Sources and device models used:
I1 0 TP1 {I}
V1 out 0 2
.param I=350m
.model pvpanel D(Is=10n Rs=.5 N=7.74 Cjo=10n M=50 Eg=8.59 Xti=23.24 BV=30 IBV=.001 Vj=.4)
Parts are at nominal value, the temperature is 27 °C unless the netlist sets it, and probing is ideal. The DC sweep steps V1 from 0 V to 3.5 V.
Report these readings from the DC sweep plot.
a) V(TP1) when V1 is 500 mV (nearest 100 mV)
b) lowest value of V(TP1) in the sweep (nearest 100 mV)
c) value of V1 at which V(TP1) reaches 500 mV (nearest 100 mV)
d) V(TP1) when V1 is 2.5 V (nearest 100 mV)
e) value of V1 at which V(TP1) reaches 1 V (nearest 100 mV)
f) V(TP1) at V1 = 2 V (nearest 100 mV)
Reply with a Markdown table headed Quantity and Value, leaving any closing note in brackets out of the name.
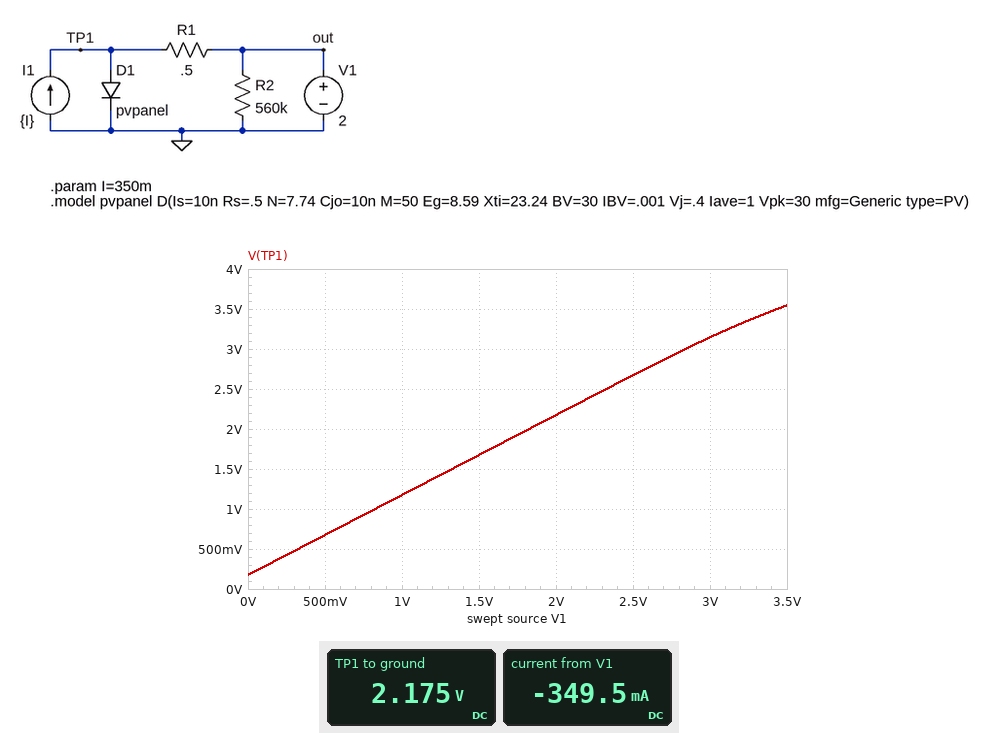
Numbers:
| Quantity | Value |
|---|---|
| V(TP1) when V1 is 500 mV | 700 mV |
| lowest value of V(TP1) in the sweep | 200 mV |
| value of V1 at which V(TP1) reaches 500 mV | 300 mV |
| V(TP1) when V1 is 2.5 V | 2.7 V |
| value of V1 at which V(TP1) reaches 1 V | 800 mV |
| V(TP1) at V1 = 2 V | 2.2 V |
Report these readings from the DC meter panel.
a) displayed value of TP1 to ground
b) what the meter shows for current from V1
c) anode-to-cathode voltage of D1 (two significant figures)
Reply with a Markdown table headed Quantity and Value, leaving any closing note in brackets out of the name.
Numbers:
| Quantity | Value |
|---|---|
| displayed value of TP1 to ground | 2.175 V |
| what the meter shows for current from V1 | -349.5 mA |
| anode-to-cathode voltage of D1 | 2.2 V |
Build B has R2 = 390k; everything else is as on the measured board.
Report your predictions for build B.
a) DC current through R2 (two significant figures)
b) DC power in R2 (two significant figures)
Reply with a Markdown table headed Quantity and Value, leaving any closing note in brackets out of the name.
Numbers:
| Quantity | Value |
|---|---|
| DC current through R2 | 5.1 µA |
| DC power in R2 | 10 µW |
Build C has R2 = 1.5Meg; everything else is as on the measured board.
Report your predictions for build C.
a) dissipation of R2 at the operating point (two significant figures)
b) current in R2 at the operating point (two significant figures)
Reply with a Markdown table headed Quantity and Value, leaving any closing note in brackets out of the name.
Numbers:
| Quantity | Value |
|---|---|
| dissipation of R2 at the operating point | 2.7 µW |
| current in R2 at the operating point | 1.3 µA |
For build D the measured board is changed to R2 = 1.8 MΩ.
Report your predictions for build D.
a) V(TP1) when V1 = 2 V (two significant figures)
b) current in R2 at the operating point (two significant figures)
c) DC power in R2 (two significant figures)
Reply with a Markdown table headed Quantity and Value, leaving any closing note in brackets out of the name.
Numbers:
| Quantity | Value |
|---|---|
| V(TP1) when V1 = 2 V | 2.2 V |
| current in R2 at the operating point | 1.1 µA |
| DC power in R2 | 2.2 µW |
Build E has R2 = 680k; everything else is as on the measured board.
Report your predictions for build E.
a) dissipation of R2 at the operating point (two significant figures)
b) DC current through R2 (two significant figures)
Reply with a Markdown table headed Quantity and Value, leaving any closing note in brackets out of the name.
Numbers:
| Quantity | Value |
|---|---|
| dissipation of R2 at the operating point | 5.9 µW |
| DC current through R2 | 2.9 µA |
